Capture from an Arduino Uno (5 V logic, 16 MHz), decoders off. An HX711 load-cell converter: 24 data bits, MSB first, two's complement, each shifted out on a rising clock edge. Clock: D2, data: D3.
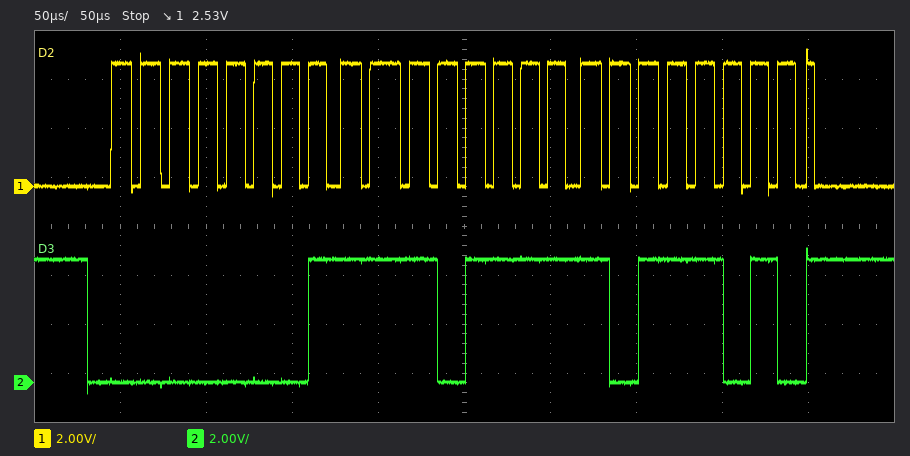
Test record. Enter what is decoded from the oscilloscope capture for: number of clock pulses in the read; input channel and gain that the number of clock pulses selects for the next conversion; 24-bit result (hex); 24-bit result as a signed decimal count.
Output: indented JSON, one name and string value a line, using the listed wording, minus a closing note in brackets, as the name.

{
  "number of clock pulses in the read": "25",
  "input channel and gain that the number of clock pulses selects for the next conversion": "channel A, gain 128",
  "24-bit result": "0x01EFBA",
  "24-bit result as a signed decimal count": "126906"
}
